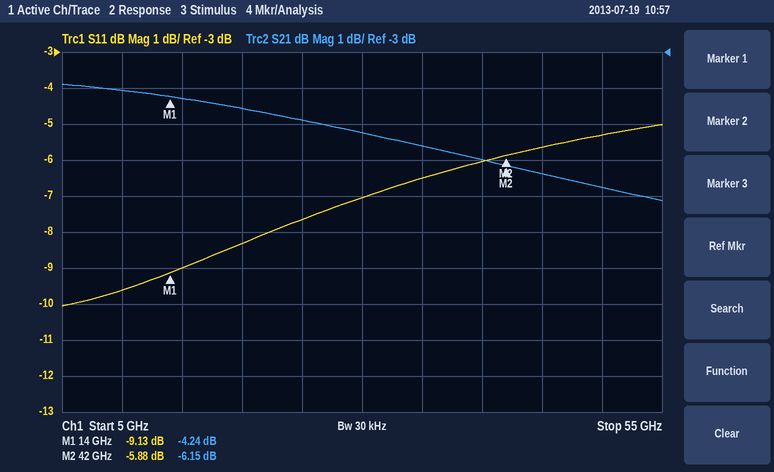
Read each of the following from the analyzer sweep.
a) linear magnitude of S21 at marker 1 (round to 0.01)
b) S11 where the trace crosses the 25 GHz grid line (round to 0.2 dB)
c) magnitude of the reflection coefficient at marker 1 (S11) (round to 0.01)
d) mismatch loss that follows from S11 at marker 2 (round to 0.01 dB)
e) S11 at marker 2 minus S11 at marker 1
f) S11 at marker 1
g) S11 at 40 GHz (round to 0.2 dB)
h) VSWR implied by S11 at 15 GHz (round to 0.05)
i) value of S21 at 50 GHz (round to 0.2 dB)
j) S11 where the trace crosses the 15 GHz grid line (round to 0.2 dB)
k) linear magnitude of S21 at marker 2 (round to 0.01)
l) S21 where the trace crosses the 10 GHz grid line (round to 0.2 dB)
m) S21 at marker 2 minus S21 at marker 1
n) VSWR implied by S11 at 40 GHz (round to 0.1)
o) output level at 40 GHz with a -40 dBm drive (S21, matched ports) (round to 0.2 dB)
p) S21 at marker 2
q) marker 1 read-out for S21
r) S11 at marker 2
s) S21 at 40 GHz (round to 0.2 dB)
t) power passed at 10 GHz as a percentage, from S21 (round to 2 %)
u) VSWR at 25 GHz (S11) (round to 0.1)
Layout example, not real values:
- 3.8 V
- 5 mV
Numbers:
- 0.61
- -7.6 dB
- 0.35
- 1.30 dB
- 3.25 dB
- -9.13 dB
- -6.0 dB
- 2.10
- -6.8 dB
- -9.0 dB
- 0.49
- -4.0 dB
- -1.91 dB
- 3.0
- -46.0 dBm
- -6.15 dB
- -4.24 dB
- -5.88 dB
- -6.0 dB
- 40 %
- 2.4
